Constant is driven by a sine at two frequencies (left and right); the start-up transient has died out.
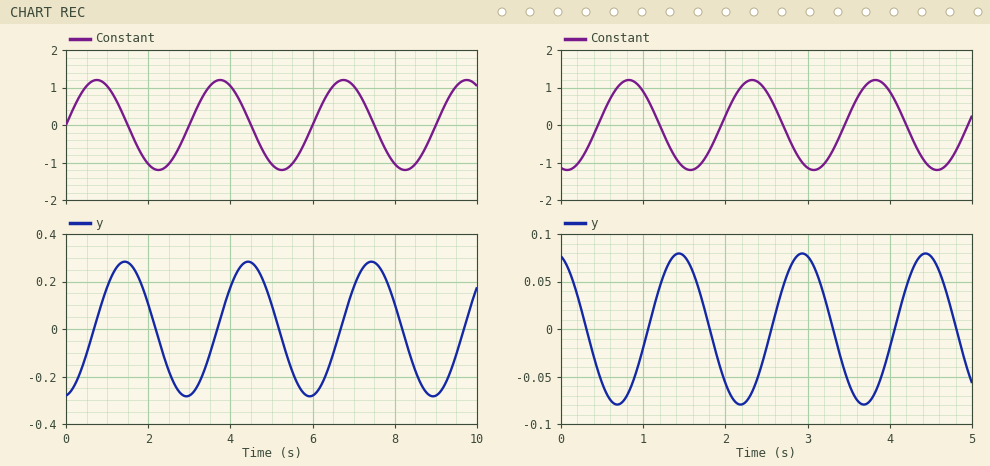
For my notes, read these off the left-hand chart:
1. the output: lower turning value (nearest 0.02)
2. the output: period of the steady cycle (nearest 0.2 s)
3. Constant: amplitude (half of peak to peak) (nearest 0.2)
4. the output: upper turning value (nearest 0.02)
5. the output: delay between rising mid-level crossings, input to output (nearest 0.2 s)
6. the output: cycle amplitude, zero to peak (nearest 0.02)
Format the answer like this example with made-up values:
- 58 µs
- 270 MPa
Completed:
- -0.28
- 3.0 s
- 1.2
- 0.28
- 0.6 s
- 0.28
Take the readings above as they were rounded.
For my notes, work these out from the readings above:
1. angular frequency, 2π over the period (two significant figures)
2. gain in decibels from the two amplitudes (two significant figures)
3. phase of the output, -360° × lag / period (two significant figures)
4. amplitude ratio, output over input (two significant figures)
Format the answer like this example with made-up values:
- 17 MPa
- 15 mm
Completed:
- 2.1 rad/s
- -13 dB
- -72°
- 0.23
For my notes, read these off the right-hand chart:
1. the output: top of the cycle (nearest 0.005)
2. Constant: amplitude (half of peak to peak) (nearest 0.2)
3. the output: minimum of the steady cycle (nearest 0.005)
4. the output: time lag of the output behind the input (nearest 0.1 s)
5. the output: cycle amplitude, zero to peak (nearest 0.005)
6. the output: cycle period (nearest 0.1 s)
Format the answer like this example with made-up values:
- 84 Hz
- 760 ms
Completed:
- 0.080
- 1.2
- -0.080
- 0.6 s
- 0.080
- 1.5 s
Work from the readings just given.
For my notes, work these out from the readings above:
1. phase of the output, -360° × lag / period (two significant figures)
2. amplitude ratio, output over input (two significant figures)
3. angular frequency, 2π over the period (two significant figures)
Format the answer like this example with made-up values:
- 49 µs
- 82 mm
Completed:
- -140°
- 0.067
- 4.2 rad/s
